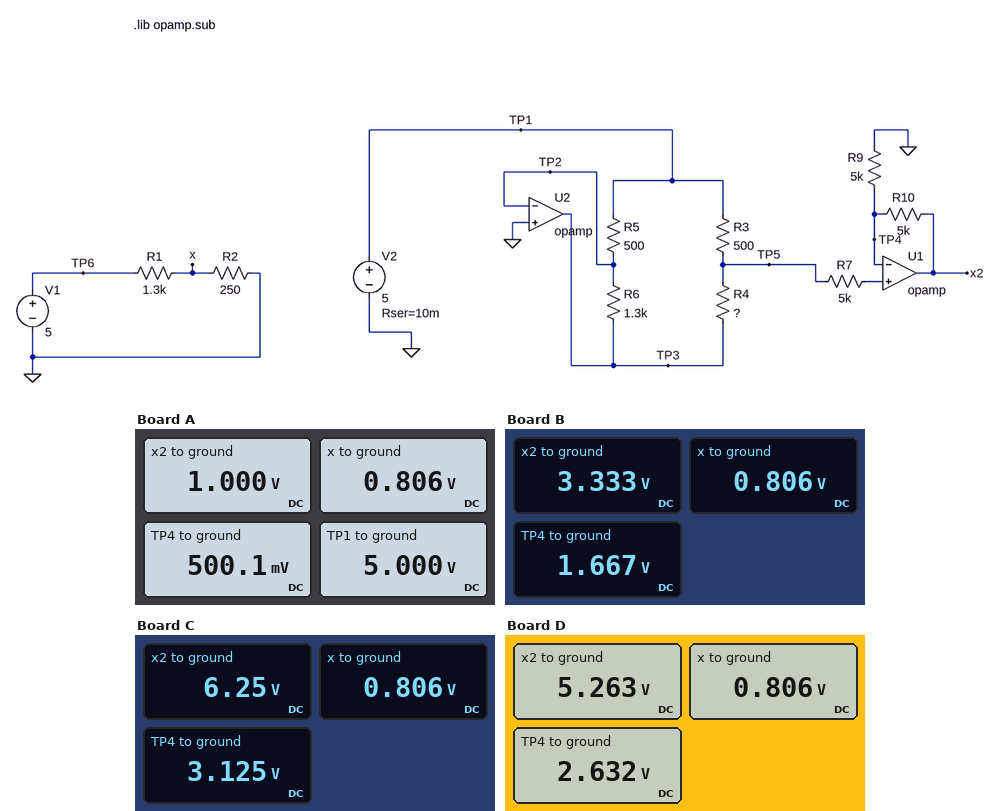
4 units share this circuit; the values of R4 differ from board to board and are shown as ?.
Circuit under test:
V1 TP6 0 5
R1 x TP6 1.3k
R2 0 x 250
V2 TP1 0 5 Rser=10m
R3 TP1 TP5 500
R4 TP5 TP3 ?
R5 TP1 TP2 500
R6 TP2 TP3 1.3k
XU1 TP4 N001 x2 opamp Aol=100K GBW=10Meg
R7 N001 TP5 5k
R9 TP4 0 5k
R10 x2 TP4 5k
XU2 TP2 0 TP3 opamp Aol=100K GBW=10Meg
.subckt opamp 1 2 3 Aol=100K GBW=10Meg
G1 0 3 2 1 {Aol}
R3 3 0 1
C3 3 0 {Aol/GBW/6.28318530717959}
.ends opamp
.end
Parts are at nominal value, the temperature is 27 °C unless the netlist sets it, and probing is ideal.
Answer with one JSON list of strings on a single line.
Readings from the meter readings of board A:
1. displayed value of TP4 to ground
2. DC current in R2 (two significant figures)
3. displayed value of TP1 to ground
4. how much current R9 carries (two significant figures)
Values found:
["500.1 mV", "3.2 mA", "5.000 V", "100 µA"]
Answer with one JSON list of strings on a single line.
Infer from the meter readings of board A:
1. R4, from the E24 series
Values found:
["1.5 kΩ"]
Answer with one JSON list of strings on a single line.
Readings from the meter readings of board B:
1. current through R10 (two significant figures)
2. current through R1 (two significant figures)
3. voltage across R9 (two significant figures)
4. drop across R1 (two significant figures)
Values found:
["330 µA", "3.2 mA", "1.7 V", "4.2 V"]
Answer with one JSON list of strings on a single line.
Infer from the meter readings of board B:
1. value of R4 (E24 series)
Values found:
["2.2 kΩ"]
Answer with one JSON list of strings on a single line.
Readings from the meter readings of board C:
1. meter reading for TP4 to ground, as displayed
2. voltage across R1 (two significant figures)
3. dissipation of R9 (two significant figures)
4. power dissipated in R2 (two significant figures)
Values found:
["3.125 V", "4.2 V", "2.0 mW", "2.6 mW"]
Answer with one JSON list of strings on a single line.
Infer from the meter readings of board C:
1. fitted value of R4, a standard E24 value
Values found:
["4.3 kΩ"]
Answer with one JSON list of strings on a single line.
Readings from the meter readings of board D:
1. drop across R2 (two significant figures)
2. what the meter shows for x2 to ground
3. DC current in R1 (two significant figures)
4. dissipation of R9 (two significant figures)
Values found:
["810 mV", "5.263 V", "3.2 mA", "1.4 mW"]
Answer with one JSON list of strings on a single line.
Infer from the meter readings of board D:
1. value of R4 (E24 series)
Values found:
["3.3 kΩ"]
